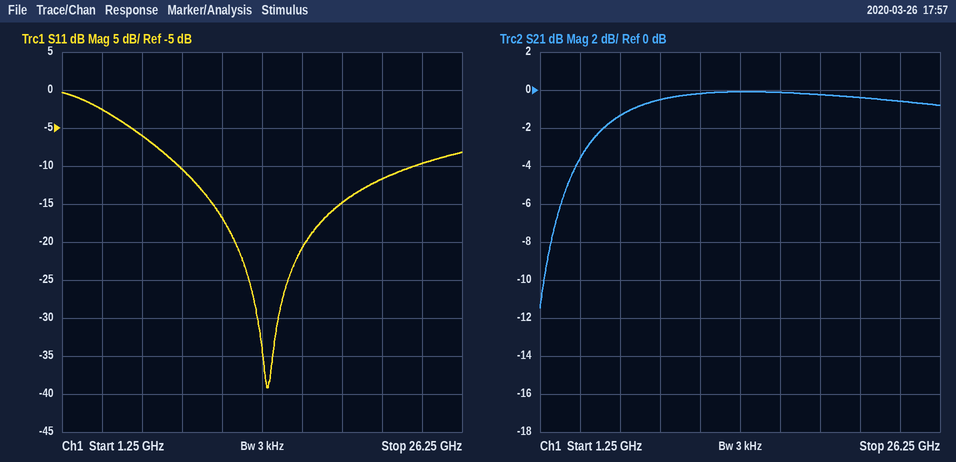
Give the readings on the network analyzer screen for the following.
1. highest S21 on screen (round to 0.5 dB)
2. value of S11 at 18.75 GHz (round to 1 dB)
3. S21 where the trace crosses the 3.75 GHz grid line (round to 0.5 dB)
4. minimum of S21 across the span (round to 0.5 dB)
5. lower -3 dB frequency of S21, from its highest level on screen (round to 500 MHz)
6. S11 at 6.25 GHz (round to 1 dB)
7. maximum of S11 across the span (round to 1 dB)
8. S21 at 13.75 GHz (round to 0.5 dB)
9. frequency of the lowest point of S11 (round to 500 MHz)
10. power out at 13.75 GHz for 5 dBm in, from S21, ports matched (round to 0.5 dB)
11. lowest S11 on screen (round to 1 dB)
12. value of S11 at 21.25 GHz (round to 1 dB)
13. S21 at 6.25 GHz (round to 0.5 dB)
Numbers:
0.0 dB
-15 dB
-3.5 dB
-11.5 dB
4.0 GHz
-6 dB
0 dB
0.0 dB
14.0 GHz
5.0 dBm
-39 dB
-12 dB
-1.5 dB
